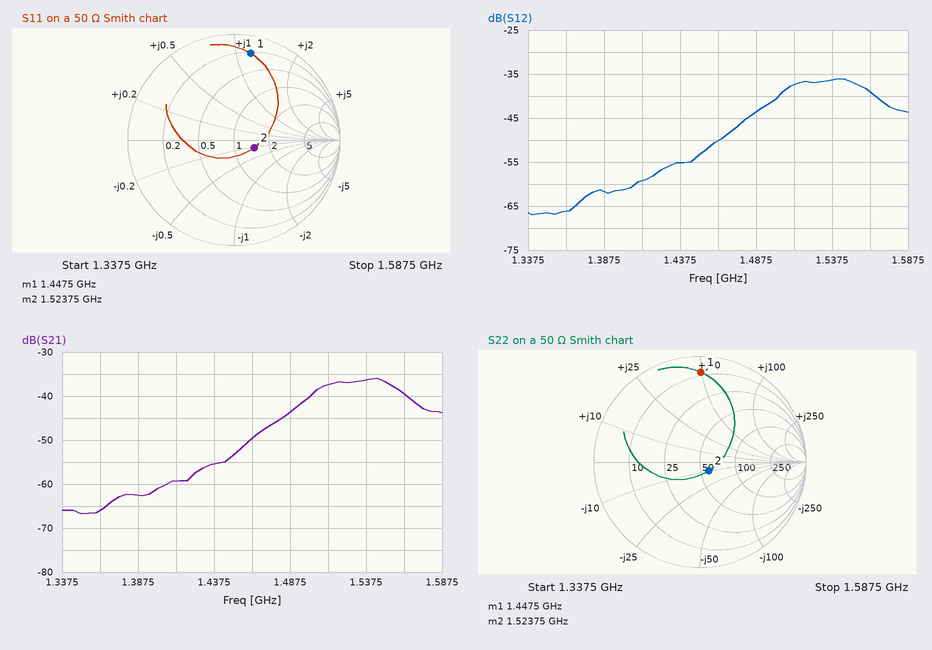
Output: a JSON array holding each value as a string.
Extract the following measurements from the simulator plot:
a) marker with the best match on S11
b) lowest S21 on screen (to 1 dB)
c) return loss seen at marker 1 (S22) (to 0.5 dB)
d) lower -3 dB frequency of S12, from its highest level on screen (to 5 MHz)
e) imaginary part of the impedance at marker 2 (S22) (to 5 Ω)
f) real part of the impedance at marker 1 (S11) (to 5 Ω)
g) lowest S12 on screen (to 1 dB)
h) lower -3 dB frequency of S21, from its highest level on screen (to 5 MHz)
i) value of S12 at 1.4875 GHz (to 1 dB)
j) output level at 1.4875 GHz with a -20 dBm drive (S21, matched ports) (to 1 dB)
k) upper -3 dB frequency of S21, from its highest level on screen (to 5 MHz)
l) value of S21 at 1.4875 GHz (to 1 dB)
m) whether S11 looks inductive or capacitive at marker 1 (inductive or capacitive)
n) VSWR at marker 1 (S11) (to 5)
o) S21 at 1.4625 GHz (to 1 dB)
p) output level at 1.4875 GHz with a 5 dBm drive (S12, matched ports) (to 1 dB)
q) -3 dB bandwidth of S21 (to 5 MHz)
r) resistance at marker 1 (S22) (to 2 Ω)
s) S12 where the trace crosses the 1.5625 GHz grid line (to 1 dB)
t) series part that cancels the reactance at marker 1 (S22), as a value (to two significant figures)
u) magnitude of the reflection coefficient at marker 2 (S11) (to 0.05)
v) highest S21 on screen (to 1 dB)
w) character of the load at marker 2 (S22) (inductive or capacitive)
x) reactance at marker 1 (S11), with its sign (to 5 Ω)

["marker 2", "-67 dB", "1.5 dB", "1.505 GHz", "-10 Ω", "10 Ω", "-67 dB", "1.505 GHz", "-44 dB", "-64 dBm", "1.560 GHz", "-44 dB", "inductive", "10", "-50 dB", "-39 dBm", "55 MHz", "8 Ω", "-39 dB", "2.2 pF", "0.20", "-36 dB", "capacitive", "+60 Ω"]
